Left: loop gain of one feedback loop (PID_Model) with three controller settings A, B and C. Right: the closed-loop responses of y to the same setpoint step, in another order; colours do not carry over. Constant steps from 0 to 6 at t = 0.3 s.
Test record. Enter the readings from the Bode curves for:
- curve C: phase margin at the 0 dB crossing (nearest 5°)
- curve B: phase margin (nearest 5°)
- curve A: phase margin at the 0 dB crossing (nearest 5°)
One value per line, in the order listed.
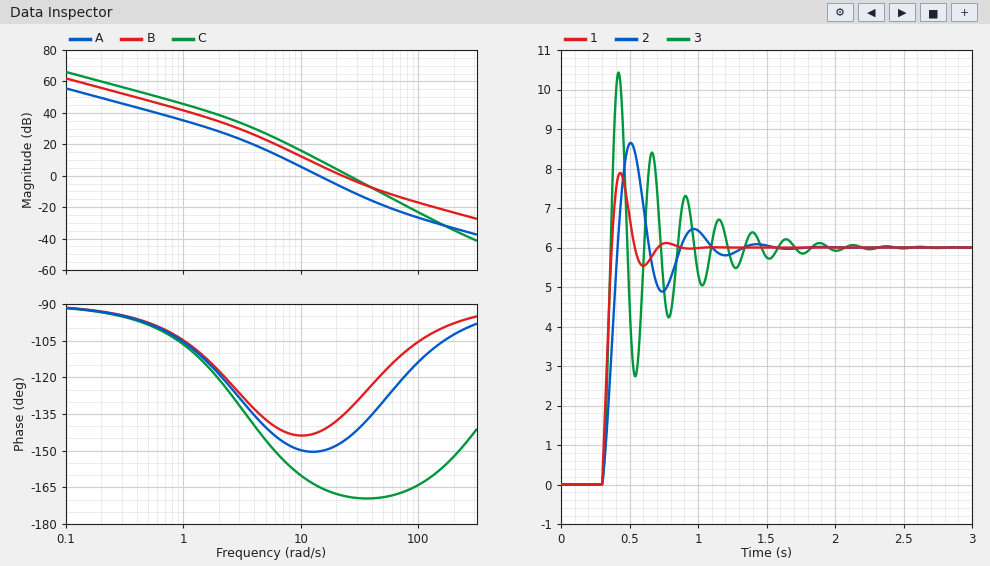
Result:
10°
45°
30°
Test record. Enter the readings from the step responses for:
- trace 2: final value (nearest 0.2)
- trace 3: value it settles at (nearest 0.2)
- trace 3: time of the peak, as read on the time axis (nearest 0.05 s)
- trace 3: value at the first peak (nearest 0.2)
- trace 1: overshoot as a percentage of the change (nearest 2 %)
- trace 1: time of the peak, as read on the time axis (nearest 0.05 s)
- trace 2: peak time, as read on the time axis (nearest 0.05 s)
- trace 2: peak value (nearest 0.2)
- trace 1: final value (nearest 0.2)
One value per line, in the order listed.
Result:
6.0
6.0
0.40 s
10.4
32 %
0.45 s
0.50 s
8.6
6.0
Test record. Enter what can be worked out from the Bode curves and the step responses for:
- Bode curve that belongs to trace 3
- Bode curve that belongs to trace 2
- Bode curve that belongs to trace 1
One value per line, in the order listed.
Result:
C
A
B
